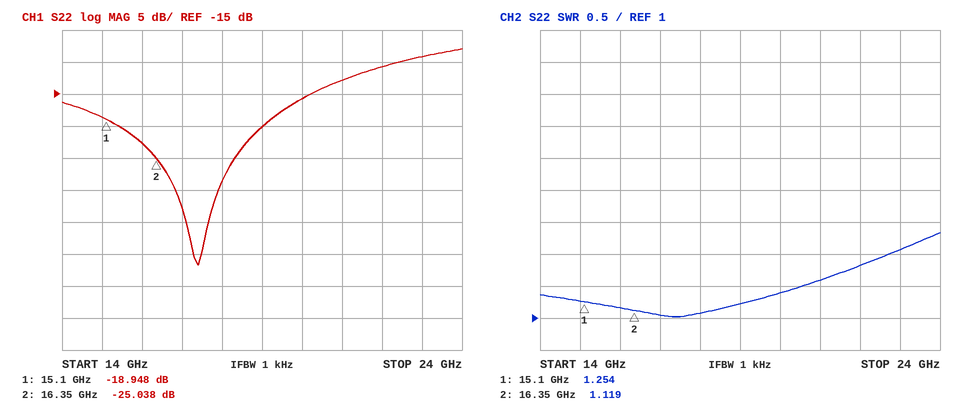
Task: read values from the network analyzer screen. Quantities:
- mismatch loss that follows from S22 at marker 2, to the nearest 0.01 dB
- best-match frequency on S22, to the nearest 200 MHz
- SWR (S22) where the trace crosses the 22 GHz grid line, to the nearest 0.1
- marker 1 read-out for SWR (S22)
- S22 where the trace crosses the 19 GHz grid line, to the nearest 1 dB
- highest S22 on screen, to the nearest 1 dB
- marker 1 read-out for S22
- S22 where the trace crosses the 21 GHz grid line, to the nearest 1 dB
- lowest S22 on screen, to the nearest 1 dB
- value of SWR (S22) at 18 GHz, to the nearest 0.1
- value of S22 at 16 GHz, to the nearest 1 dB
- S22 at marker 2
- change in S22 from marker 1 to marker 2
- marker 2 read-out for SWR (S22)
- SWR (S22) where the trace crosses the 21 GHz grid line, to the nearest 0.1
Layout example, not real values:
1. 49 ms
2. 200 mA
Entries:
1. 0.01 dB
2. 17.4 GHz
3. 1.8
4. 1.254
5. -20 dB
6. -8 dB
7. -18.948 dB
8. -13 dB
9. -42 dB
10. 1.1
11. -23 dB
12. -25.038 dB
13. -6.090 dB
14. 1.119
15. 1.6
